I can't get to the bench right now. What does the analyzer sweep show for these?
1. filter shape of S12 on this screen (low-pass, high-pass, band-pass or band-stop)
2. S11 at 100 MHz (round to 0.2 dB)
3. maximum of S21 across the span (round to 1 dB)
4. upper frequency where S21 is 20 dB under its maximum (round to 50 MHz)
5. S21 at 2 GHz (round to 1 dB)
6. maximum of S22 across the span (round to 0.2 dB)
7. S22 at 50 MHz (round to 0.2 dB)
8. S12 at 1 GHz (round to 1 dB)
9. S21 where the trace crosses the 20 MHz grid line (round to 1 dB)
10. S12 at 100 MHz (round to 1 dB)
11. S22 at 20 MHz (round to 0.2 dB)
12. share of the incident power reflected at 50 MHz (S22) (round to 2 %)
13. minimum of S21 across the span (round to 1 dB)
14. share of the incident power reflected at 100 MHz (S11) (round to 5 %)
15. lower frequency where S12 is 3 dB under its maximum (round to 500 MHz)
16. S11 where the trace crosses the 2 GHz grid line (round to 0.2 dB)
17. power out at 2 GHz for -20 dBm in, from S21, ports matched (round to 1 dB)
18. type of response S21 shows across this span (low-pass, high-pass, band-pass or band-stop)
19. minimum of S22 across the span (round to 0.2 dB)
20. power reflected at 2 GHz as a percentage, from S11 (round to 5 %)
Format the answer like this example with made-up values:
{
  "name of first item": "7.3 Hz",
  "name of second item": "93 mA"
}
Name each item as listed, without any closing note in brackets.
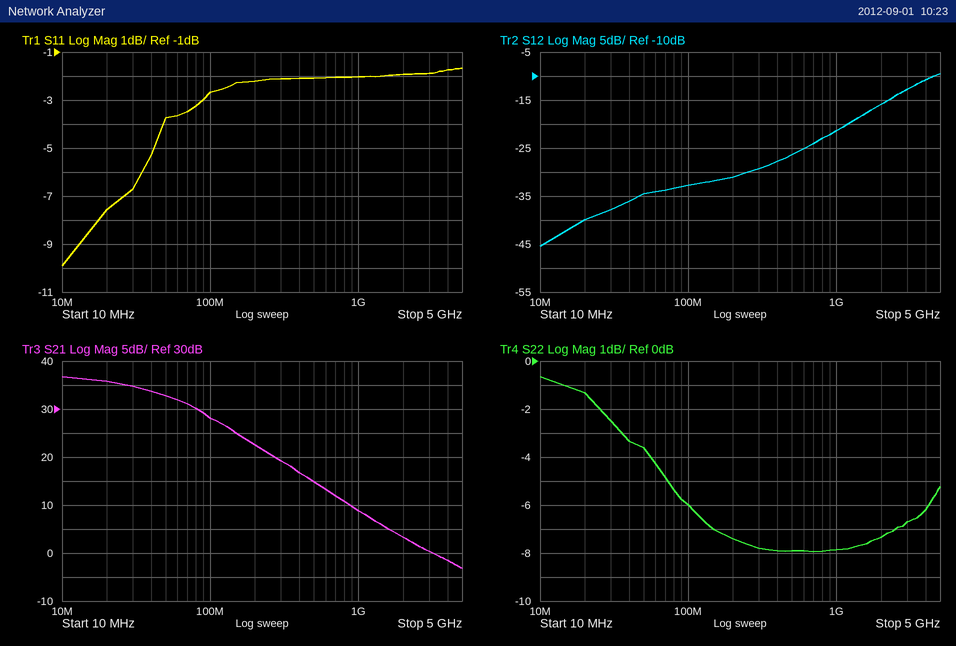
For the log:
{
  "filter shape of S12 on this screen": "high-pass",
  "S11 at 100 MHz": "-2.6 dB",
  "maximum of S21 across the span": "37 dB",
  "upper frequency where S21 is 20 dB under its maximum": "400 MHz",
  "S21 at 2 GHz": "3 dB",
  "maximum of S22 across the span": "-0.6 dB",
  "S22 at 50 MHz": "-3.6 dB",
  "S12 at 1 GHz": "-21 dB",
  "S21 where the trace crosses the 20 MHz grid line": "36 dB",
  "S12 at 100 MHz": "-33 dB",
  "S22 at 20 MHz": "-1.4 dB",
  "share of the incident power reflected at 50 MHz (S22)": "44 %",
  "minimum of S21 across the span": "-3 dB",
  "share of the incident power reflected at 100 MHz (S11)": "55 %",
  "lower frequency where S12 is 3 dB under its maximum": "3.0 GHz",
  "S11 where the trace crosses the 2 GHz grid line": "-2.0 dB",
  "power out at 2 GHz for -20 dBm in, from S21, ports matched": "-17 dBm",
  "type of response S21 shows across this span": "low-pass",
  "minimum of S22 across the span": "-8.0 dB",
  "power reflected at 2 GHz as a percentage, from S11": "65 %"
}
